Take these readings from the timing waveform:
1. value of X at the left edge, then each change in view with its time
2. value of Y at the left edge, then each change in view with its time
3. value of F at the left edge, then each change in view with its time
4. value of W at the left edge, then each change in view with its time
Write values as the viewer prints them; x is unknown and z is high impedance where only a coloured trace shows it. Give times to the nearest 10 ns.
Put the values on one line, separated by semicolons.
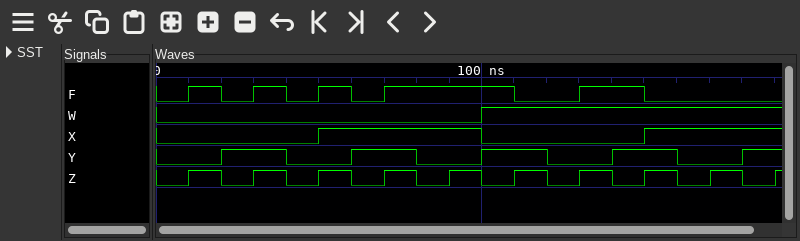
0, 1 at 50 ns, 0 at 100 ns, 1 at 150 ns; 0, 1 at 20 ns, 0 at 40 ns, 1 at 60 ns, 0 at 80 ns, 1 at 100 ns, 0 at 120 ns, 1 at 140 ns, 0 at 160 ns, 1 at 180 ns; 0, 1 at 10 ns, 0 at 20 ns, 1 at 30 ns, 0 at 40 ns, 1 at 50 ns, 0 at 60 ns, 1 at 70 ns, 0 at 110 ns, 1 at 130 ns, 0 at 150 ns; 0, 1 at 100 ns
